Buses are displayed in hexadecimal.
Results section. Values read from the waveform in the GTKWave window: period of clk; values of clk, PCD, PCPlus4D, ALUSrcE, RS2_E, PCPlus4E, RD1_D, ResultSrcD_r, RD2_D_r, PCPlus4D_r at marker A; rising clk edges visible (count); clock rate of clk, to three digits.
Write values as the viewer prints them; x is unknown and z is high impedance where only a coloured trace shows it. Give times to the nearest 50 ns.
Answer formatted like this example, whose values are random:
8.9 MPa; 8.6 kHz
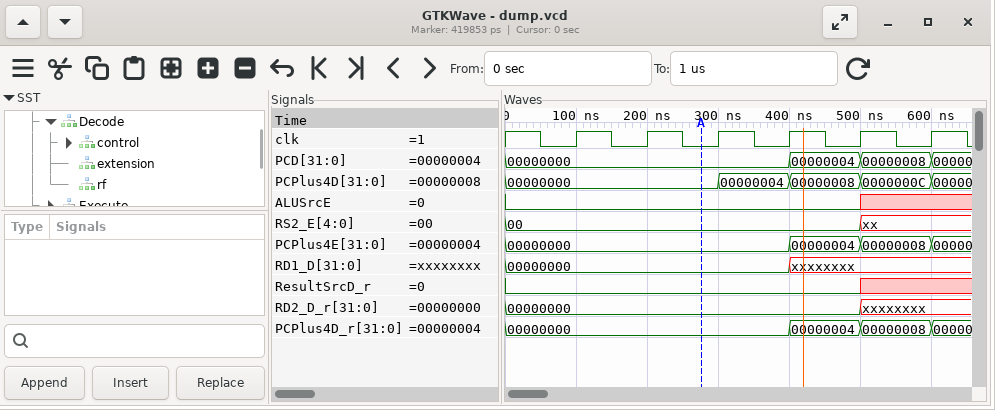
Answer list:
100 ns; clk=0, PCD=00000000, PCPlus4D=00000000, ALUSrcE=0, RS2_E=00, PCPlus4E=00000000, RD1_D=00000000, ResultSrcD_r=0, RD2_D_r=00000000, PCPlus4D_r=00000000; 6; 10.0 MHz
